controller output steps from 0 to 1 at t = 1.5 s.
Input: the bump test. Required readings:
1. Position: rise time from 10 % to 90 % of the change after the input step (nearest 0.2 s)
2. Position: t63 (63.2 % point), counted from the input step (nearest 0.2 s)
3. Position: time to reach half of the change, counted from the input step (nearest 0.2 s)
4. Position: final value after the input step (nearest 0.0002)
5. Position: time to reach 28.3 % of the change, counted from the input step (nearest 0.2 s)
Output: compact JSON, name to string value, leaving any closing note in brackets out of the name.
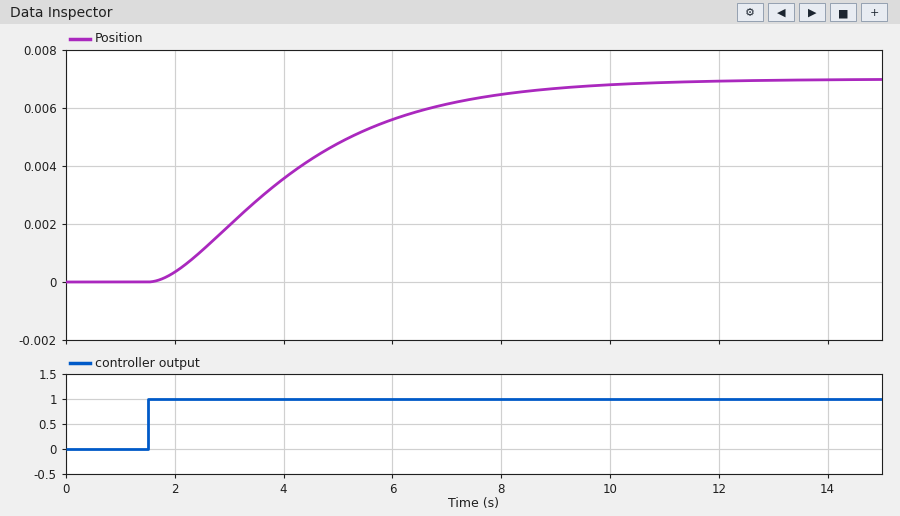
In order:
{"Position: rise time from 10 % to 90 % of the change after the input step": "5.2 s", "Position: t63 (63.2 % point), counted from the input step": "3.2 s", "Position: time to reach half of the change, counted from the input step": "2.4 s", "Position: final value after the input step": "0.0070", "Position: time to reach 28.3 % of the change, counted from the input step": "1.6 s"}
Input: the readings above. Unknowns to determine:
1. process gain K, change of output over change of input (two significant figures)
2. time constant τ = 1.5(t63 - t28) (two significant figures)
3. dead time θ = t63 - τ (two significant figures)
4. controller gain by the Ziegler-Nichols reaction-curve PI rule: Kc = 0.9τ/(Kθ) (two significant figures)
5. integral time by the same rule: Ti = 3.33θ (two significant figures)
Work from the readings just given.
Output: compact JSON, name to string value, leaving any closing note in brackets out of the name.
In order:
{"process gain K, change of output over change of input": "0.0070", "time constant τ = 1.5(t63 - t28)": "2.4 s", "dead time θ = t63 - τ": "0.80 s", "controller gain by the Ziegler-Nichols reaction-curve PI rule: Kc = 0.9τ/(Kθ)": "390", "integral time by the same rule: Ti = 3.33θ": "2.7 s"}
